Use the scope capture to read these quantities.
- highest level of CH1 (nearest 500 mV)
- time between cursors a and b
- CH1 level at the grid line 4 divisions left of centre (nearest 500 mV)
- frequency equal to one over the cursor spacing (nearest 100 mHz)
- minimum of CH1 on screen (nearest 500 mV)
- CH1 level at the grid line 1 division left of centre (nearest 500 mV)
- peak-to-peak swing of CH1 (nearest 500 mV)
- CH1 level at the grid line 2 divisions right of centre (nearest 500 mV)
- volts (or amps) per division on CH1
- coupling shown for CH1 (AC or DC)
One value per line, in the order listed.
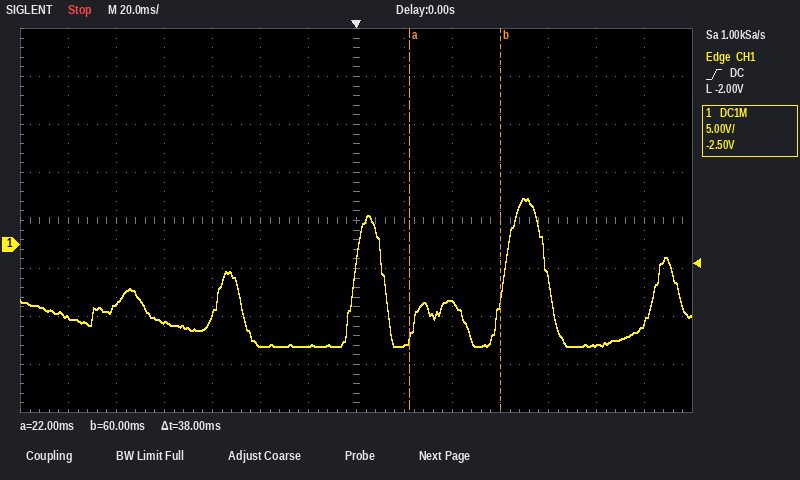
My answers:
5.0 V
38 ms
-8.0 V
26.3 Hz
-10.5 V
-10.5 V
15.5 V
-6.0 V
5 V
DC
